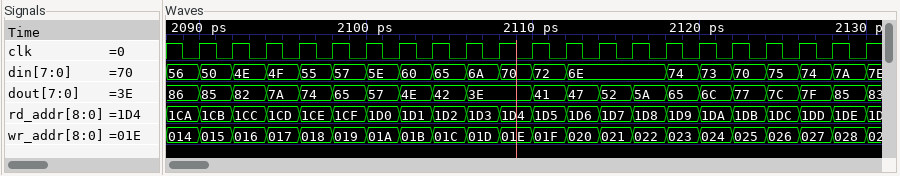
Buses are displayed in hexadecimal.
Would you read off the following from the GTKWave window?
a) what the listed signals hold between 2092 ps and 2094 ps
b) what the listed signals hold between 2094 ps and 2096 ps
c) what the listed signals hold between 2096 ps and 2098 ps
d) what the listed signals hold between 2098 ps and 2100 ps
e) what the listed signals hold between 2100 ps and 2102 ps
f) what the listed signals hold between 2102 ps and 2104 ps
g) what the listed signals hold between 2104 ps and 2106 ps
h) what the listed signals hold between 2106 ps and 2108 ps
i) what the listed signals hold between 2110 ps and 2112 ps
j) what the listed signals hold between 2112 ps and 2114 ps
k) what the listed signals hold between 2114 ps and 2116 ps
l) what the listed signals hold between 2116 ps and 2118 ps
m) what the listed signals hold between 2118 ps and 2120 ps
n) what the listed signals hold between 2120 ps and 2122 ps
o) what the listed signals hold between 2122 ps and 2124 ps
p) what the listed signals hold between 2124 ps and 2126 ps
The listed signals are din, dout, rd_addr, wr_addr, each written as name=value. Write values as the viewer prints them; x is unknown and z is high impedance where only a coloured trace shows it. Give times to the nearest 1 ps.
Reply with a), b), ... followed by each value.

a) din=4E, dout=82, rd_addr=1CC, wr_addr=016
b) din=4F, dout=7A, rd_addr=1CD, wr_addr=017
c) din=55, dout=74, rd_addr=1CE, wr_addr=018
d) din=57, dout=65, rd_addr=1CF, wr_addr=019
e) din=5E, dout=57, rd_addr=1D0, wr_addr=01A
f) din=60, dout=4E, rd_addr=1D1, wr_addr=01B
g) din=65, dout=42, rd_addr=1D2, wr_addr=01C
h) din=6A, dout=3E, rd_addr=1D3, wr_addr=01D
i) din=72, dout=41, rd_addr=1D5, wr_addr=01F
j) din=6E, dout=47, rd_addr=1D6, wr_addr=020
k) din=6E, dout=52, rd_addr=1D7, wr_addr=021
l) din=6E, dout=5A, rd_addr=1D8, wr_addr=022
m) din=74, dout=65, rd_addr=1D9, wr_addr=023
n) din=73, dout=6C, rd_addr=1DA, wr_addr=024
o) din=70, dout=77, rd_addr=1DB, wr_addr=025
p) din=75, dout=7C, rd_addr=1DC, wr_addr=026
